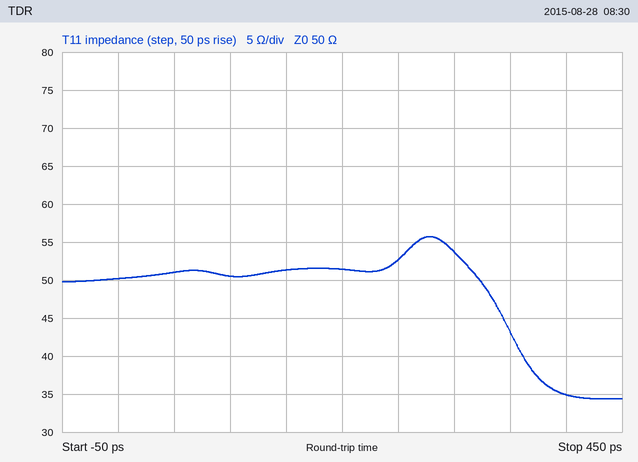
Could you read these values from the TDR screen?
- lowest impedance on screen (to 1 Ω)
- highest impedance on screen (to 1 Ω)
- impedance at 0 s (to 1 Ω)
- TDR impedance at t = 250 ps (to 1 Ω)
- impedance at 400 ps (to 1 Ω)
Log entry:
34 Ω
56 Ω
50 Ω
53 Ω
35 Ω
